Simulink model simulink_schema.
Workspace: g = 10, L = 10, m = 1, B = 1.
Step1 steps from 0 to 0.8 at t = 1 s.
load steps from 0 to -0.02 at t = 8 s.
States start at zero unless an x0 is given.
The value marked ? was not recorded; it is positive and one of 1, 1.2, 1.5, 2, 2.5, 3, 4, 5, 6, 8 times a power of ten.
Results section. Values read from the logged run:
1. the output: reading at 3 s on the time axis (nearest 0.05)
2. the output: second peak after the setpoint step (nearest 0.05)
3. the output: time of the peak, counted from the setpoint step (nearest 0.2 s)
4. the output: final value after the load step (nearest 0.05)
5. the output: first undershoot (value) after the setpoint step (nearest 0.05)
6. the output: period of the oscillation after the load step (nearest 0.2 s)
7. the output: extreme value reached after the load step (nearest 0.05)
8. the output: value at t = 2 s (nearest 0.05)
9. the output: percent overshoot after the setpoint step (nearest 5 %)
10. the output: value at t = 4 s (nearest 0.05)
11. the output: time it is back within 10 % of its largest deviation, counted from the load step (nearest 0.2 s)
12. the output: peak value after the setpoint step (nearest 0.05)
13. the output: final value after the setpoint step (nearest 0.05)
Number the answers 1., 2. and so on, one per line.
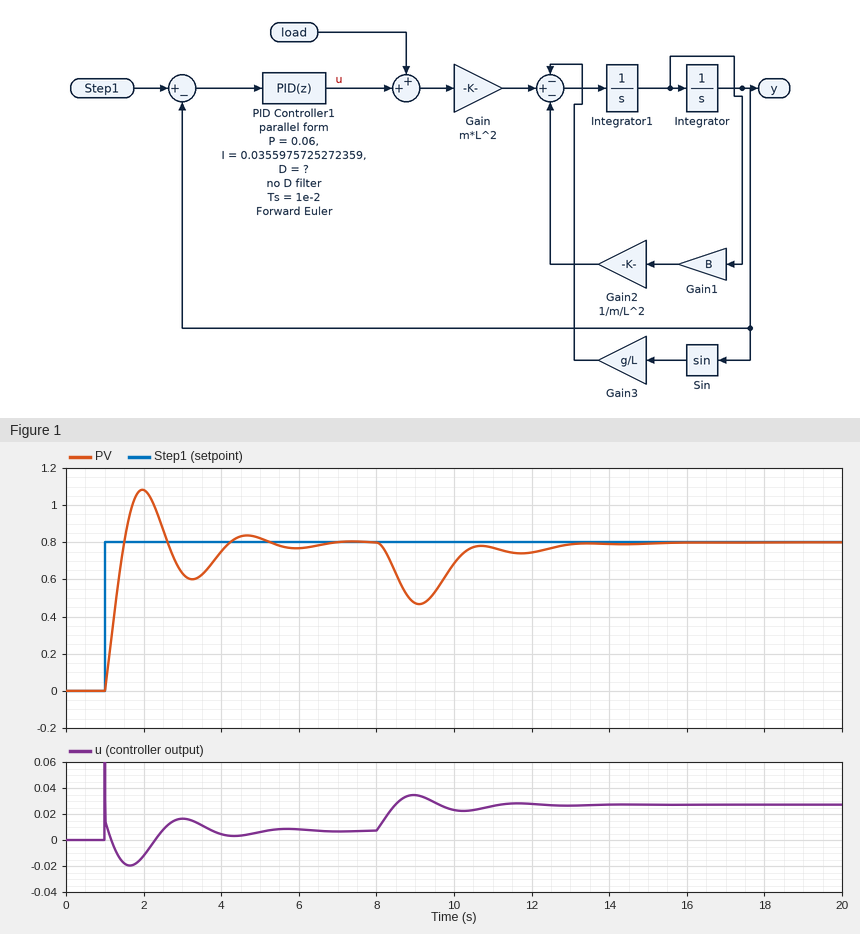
1. 0.65
2. 0.85
3. 1.0 s
4. 0.80
5. 0.60
6. 2.6 s
7. 0.45
8. 1.10
9. 35 %
10. 0.75
11. 4.4 s
12. 1.10
13. 0.80
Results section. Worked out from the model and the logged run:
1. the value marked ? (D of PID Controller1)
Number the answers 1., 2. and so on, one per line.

1. 0.02
